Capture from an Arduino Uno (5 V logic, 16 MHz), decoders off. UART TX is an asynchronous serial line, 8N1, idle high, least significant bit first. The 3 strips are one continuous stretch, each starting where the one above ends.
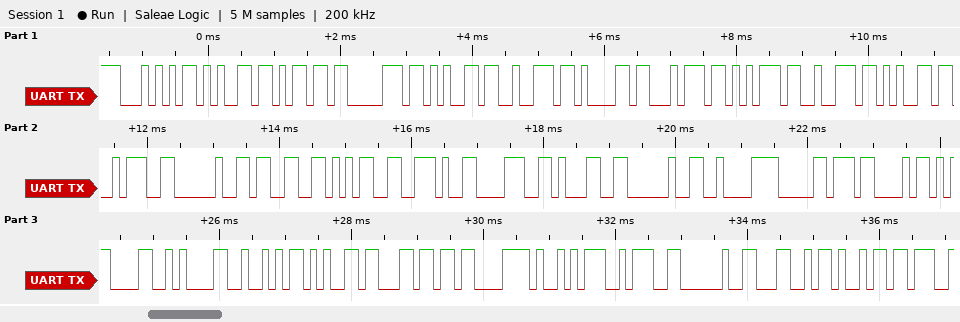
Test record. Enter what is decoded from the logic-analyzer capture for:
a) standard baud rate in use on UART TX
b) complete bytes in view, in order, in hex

9600 baud
54 65 6D 70 65 72 61 74 75 72 65 3A 20 33 35 2E 38 31 20 C2 B0 43 0D 0A 52 65 6C C3 A9 3A 20 4C 69
